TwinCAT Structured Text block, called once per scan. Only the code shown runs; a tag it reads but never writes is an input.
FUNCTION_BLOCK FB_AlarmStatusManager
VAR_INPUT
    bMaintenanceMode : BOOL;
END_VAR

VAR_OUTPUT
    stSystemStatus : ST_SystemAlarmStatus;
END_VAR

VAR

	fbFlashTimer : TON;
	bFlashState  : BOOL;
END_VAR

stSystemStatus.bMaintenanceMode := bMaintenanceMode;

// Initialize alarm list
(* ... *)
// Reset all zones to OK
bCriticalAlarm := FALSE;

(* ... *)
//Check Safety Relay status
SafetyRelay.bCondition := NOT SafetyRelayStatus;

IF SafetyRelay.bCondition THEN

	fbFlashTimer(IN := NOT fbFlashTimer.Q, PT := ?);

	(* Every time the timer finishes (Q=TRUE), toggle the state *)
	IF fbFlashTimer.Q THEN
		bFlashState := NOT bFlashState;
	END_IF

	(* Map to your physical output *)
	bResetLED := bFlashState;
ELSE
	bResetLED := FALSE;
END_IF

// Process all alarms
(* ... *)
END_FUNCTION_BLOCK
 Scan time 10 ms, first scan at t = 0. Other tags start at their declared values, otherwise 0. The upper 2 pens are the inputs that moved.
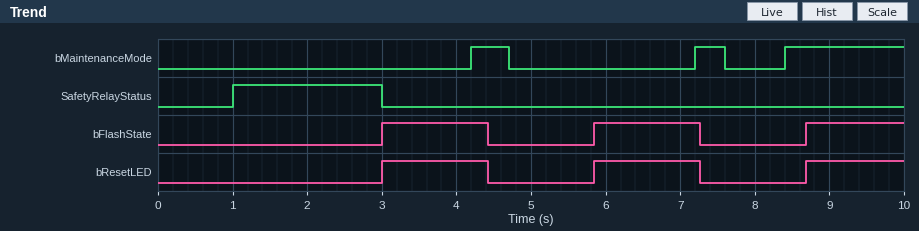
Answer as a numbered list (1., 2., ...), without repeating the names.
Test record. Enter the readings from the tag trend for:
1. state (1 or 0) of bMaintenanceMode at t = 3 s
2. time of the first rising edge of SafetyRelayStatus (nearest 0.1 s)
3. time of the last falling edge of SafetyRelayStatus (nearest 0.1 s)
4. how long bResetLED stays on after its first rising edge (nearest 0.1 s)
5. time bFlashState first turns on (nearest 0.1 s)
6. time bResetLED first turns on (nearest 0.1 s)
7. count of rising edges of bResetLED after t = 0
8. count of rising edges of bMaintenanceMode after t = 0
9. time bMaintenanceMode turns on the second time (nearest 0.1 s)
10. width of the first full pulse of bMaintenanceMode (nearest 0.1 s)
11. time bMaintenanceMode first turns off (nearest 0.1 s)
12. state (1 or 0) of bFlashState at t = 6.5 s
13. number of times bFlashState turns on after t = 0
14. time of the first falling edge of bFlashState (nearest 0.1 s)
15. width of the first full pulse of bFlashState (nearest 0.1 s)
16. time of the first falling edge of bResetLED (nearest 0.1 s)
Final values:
1. 0
2. 1.0 s
3. 3.0 s
4. 1.4 s
5. 3.0 s
6. 3.0 s
7. 3
8. 3
9. 7.2 s
10. 0.5 s
11. 4.7 s
12. 1
13. 3
14. 4.4 s
15. 1.4 s
16. 4.4 s
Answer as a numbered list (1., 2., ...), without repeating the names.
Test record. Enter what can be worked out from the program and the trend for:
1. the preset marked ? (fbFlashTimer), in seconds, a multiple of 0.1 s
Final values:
1. 1.4 s
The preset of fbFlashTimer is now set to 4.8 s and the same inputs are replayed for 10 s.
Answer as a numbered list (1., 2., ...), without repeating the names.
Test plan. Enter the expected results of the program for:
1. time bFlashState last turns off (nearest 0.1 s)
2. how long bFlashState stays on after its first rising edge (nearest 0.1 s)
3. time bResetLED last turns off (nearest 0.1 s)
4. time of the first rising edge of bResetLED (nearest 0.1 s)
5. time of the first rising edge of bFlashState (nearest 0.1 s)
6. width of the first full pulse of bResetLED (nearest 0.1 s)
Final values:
1. 9.6 s
2. 4.8 s
3. 9.6 s
4. 4.8 s
5. 4.8 s
6. 4.8 s
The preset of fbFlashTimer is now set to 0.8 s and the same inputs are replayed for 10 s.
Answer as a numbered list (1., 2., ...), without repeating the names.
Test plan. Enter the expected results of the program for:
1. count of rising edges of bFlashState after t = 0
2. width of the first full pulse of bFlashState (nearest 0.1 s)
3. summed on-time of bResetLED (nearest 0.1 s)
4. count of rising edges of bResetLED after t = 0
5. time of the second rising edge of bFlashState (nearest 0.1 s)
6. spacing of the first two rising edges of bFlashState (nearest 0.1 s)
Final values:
1. 5
2. 2.2 s
3. 3.5 s
4. 5
5. 3.8 s
6. 3.0 s
